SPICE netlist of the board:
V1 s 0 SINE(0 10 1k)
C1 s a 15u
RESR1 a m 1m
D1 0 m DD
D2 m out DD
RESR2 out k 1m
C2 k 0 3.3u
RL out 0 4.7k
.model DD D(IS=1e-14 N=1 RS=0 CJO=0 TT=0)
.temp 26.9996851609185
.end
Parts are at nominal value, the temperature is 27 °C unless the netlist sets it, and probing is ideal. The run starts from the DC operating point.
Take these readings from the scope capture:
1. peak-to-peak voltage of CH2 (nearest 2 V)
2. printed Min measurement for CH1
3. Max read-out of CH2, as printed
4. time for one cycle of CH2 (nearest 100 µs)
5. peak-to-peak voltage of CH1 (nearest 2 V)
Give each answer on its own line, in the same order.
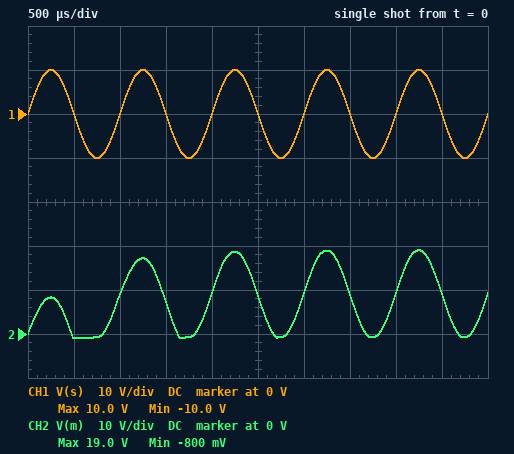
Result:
20 V
-10.0 V
19.0 V
1.0 ms
20 V
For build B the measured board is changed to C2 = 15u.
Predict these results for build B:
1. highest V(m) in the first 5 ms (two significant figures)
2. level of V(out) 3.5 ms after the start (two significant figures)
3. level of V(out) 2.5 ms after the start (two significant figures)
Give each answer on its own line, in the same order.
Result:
18 V
17 V
15 V
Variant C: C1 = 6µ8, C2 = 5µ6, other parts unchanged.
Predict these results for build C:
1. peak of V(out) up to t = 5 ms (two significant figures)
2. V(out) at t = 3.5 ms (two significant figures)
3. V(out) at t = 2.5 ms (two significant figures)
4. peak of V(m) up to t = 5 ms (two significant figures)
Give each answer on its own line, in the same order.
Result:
18 V
17 V
15 V
18 V
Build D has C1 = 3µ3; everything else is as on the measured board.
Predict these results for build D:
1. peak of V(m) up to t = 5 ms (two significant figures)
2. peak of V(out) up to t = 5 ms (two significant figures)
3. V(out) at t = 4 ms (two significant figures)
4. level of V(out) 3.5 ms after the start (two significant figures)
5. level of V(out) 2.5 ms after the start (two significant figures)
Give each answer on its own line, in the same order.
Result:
18 V
17 V
15 V
16 V
14 V
